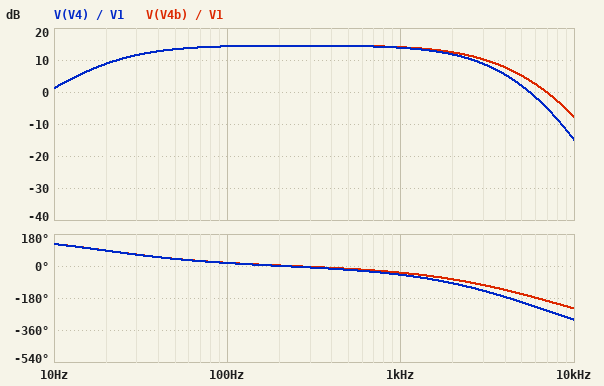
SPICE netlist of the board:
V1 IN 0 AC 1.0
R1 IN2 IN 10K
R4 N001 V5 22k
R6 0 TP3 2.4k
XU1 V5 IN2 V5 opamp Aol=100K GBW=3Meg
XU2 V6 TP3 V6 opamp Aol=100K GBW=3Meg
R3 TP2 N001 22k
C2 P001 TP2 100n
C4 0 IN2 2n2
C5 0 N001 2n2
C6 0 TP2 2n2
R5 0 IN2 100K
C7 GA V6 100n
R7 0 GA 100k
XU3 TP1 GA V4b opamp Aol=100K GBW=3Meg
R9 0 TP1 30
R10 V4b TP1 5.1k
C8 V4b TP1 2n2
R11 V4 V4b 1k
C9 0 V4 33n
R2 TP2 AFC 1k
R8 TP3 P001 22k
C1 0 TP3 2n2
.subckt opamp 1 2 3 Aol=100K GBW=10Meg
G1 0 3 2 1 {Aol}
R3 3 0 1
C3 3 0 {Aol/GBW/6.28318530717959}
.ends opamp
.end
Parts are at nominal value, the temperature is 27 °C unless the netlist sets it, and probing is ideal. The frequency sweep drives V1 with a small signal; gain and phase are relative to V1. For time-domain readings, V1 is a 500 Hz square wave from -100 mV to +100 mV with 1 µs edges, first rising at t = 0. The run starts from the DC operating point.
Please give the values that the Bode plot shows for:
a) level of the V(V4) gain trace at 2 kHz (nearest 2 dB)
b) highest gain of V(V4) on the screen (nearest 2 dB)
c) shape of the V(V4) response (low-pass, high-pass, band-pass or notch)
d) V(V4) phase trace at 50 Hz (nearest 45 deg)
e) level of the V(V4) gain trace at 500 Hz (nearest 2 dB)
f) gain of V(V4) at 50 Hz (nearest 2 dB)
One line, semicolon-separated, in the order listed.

12 dB; 14 dB; band-pass; 45 deg; 14 dB; 14 dB
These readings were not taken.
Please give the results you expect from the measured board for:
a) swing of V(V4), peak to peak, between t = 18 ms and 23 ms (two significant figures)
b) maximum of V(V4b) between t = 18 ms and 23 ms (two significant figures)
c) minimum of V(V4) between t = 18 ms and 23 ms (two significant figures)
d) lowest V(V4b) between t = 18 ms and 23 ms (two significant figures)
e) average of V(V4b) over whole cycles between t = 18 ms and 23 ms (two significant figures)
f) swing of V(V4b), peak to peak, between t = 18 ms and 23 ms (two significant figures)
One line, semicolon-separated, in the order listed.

1.1 V; 510 mV; -630 mV; -630 mV; -65 mV; 1.1 V
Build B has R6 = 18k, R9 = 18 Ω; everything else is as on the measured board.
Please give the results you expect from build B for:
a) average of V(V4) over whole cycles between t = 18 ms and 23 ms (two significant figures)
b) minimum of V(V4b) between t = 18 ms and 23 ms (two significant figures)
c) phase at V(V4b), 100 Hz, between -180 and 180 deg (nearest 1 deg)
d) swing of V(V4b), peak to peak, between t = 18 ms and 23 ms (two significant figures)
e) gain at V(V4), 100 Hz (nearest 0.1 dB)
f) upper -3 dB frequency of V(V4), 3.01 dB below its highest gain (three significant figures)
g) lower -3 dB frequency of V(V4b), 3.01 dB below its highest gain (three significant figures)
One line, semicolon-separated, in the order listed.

-720 mV; -6.3 V; 14 deg; 11 V; 34.5 dB; 1.58 kHz; 26.4 Hz
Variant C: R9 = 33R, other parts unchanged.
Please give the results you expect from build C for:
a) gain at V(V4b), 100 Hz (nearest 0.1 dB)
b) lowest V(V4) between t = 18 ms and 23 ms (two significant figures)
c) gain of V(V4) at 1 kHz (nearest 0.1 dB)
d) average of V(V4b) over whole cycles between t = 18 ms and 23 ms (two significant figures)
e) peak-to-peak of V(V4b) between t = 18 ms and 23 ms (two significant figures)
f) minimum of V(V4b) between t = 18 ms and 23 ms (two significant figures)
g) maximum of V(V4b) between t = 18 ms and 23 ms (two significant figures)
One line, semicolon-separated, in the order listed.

13.5 dB; -570 mV; 13.0 dB; -59 mV; 1.0 V; -580 mV; 460 mV
